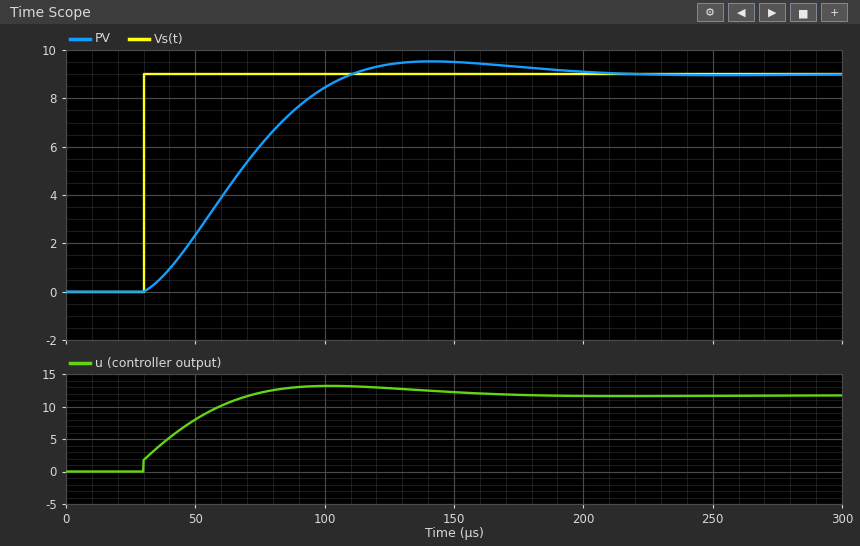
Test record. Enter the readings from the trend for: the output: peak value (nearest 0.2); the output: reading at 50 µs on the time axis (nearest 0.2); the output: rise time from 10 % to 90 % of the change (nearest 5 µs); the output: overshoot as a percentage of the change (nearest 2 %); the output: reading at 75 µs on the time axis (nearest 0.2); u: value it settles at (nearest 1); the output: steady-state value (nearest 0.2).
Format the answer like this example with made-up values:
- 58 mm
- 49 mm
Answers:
- 9.6
- 2.4
- 55 µs
- 6 %
- 6.0
- 12
- 9.0
